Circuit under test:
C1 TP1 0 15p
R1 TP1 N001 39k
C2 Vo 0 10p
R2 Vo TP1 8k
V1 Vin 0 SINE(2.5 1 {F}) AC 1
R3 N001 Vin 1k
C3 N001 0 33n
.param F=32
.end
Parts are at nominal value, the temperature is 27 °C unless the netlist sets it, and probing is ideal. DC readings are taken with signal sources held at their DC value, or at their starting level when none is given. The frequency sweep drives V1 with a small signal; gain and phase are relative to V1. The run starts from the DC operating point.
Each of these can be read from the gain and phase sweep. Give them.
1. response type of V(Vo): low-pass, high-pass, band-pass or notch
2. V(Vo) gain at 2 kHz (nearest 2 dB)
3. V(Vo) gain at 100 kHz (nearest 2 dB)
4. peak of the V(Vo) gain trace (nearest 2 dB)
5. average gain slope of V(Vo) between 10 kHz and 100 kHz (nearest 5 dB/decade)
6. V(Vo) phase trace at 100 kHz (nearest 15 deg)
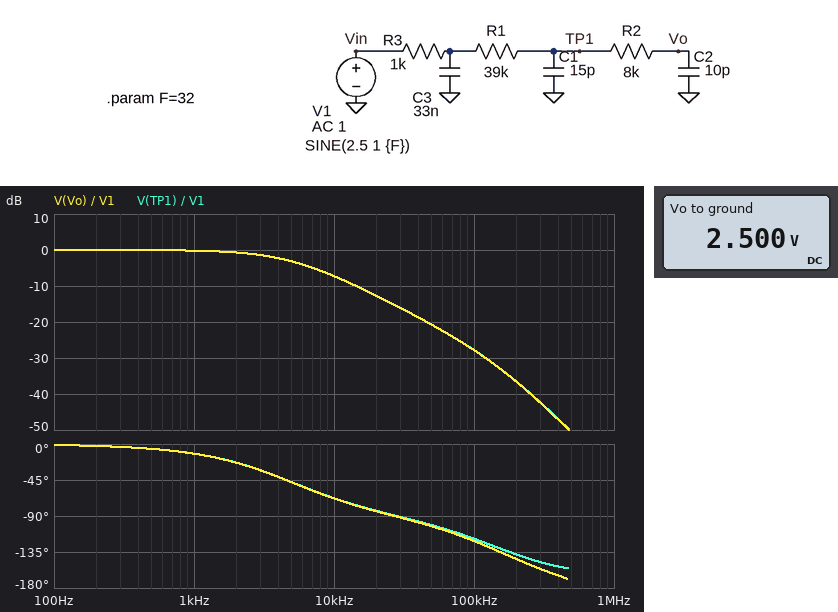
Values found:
low-pass
0 dB
-28 dB
0 dB
-20 dB/decade
-120 deg
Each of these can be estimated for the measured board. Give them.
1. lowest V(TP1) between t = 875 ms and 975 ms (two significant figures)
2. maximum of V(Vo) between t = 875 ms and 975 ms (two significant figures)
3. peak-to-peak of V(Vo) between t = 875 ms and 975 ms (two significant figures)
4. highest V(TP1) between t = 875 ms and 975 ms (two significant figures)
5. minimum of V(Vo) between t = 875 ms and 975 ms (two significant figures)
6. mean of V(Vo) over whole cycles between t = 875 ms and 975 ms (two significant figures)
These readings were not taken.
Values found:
1.5 V
3.5 V
2.0 V
3.5 V
1.5 V
2.5 V
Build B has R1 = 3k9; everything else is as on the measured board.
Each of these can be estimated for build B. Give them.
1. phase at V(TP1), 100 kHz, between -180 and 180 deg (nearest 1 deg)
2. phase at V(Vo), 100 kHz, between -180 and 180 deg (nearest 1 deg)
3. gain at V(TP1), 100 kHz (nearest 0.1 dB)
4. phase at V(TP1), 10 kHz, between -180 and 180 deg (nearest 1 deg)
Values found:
-91 deg
-94 deg
-26.4 dB
-65 deg
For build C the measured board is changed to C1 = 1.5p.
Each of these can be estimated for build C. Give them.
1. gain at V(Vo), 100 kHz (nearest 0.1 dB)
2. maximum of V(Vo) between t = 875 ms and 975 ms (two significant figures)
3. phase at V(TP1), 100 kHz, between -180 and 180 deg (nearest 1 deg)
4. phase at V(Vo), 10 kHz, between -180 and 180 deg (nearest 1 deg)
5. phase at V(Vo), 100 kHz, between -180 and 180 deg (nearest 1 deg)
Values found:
-26.8 dB
3.5 V
-103 deg
-66 deg
-106 deg
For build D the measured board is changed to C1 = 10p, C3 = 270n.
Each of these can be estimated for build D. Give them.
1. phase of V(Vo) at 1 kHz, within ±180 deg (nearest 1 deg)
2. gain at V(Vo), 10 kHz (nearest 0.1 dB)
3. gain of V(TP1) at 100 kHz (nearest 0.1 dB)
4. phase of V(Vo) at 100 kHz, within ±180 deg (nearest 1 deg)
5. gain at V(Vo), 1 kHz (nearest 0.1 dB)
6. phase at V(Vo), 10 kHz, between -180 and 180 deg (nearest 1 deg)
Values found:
-60 deg
-24.6 dB
-45.6 dB
-118 deg
-5.9 dB
-90 deg
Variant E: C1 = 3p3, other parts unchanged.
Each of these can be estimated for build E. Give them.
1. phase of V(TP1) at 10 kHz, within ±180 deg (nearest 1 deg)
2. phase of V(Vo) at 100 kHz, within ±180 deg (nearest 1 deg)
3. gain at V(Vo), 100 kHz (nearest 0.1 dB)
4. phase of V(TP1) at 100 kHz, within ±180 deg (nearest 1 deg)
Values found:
-66 deg
-108 deg
-26.9 dB
-105 deg
